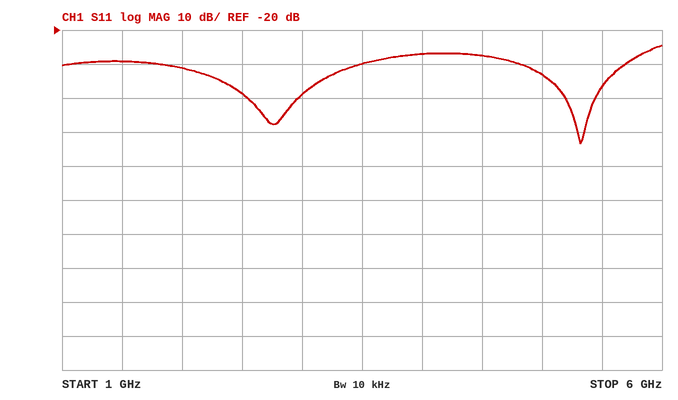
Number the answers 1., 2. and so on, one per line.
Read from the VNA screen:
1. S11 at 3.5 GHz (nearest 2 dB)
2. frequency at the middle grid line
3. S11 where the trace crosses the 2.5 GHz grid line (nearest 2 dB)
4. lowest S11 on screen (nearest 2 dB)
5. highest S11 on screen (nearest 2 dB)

1. -30 dB
2. 3.5 GHz
3. -38 dB
4. -54 dB
5. -24 dB
